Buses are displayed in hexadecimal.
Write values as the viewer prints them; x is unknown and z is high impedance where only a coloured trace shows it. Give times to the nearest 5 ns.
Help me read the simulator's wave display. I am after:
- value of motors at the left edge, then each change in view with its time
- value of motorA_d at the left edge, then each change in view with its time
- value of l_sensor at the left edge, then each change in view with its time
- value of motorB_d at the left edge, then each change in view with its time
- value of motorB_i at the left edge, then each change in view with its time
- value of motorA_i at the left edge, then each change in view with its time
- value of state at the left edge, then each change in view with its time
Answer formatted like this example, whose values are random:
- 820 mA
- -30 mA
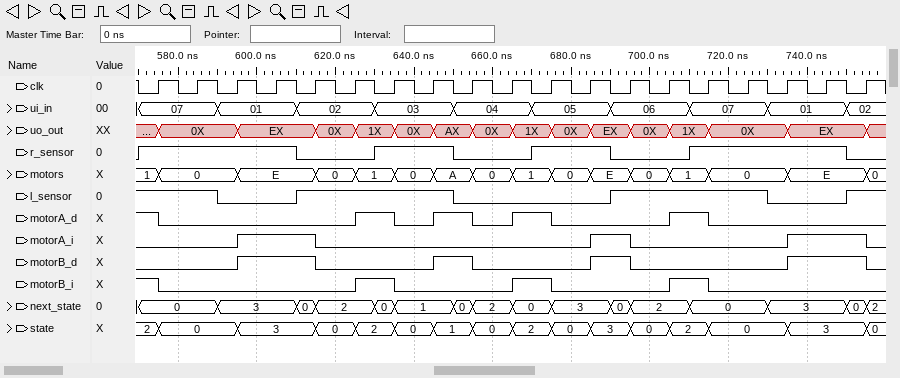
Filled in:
- 1, 0 at 575 ns, E at 595 ns, 0 at 615 ns, 1 at 625 ns, 0 at 635 ns, A at 645 ns, 0 at 655 ns, 1 at 665 ns, 0 at 675 ns, E at 685 ns, 0 at 695 ns, 1 at 705 ns, 0 at 715 ns, E at 735 ns, 0 at 755 ns
- 1, 0 at 575 ns, 1 at 625 ns, 0 at 635 ns, 1 at 645 ns, 0 at 655 ns, 1 at 665 ns, 0 at 675 ns, 1 at 705 ns, 0 at 715 ns
- 1, 0 at 590 ns, 1 at 610 ns, 0 at 650 ns, 1 at 690 ns, 0 at 730 ns, 1 at 750 ns
- 0, 1 at 595 ns, 0 at 615 ns, 1 at 645 ns, 0 at 655 ns, 1 at 685 ns, 0 at 695 ns, 1 at 735 ns, 0 at 755 ns
- 1, 0 at 575 ns, 1 at 625 ns, 0 at 635 ns, 1 at 665 ns, 0 at 675 ns, 1 at 705 ns, 0 at 715 ns
- 0, 1 at 595 ns, 0 at 615 ns, 1 at 685 ns, 0 at 695 ns, 1 at 735 ns, 0 at 755 ns
- 2, 0 at 575 ns, 3 at 595 ns, 0 at 615 ns, 2 at 625 ns, 0 at 635 ns, 1 at 645 ns, 0 at 655 ns, 2 at 665 ns, 0 at 675 ns, 3 at 685 ns, 0 at 695 ns, 2 at 705 ns, 0 at 715 ns, 3 at 735 ns, 0 at 755 ns
